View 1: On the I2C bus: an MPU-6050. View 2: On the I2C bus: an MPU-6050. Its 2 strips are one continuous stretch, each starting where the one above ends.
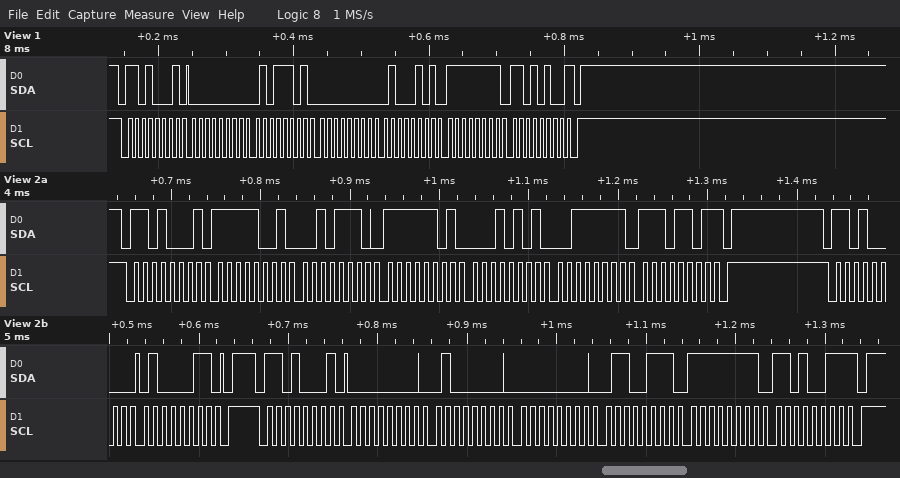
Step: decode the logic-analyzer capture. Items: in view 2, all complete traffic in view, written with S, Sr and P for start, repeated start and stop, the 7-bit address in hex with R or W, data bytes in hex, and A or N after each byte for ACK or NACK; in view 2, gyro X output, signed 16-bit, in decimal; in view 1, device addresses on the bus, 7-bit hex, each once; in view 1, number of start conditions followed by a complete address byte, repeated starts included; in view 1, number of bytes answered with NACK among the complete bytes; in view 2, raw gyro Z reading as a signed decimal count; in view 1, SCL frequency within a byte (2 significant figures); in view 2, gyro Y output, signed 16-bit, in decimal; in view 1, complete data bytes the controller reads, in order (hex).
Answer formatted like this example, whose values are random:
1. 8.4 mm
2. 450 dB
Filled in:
1. S 68R A F9 A 2E A FD A 15 A 3F A ED N P S 68W A 43 A P S 68R A 00 A 40 A 00 A 67 A FF A D3 N P
2. 64
3. 0x68
4. 1
5. 1
6. -45
7. 100 kHz
8. 103
9. 00 5D 00 45 FF D4
